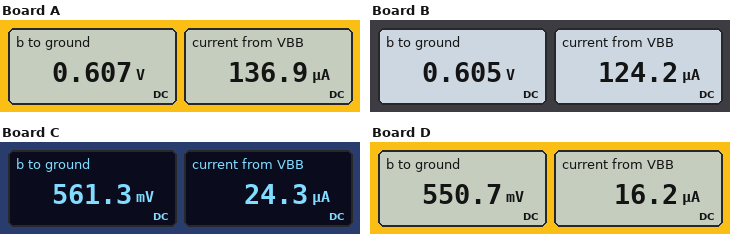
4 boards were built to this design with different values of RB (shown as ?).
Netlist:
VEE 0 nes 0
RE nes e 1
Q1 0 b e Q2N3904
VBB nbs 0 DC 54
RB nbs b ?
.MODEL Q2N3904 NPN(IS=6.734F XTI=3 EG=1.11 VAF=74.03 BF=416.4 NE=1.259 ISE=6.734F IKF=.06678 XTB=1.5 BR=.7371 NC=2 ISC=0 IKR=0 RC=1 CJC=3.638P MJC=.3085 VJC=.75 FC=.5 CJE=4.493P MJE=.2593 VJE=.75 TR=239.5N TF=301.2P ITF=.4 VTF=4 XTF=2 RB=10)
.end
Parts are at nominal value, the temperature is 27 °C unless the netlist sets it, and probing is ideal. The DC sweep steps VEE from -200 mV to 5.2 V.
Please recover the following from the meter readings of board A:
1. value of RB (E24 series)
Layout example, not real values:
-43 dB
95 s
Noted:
390 kΩ
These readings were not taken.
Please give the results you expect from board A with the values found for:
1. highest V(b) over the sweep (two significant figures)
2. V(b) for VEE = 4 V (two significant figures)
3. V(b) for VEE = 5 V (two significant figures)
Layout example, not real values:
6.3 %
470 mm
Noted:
610 mV
-3.2 V
-4.2 V
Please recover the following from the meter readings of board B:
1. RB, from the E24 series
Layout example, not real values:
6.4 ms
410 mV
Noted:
430 kΩ
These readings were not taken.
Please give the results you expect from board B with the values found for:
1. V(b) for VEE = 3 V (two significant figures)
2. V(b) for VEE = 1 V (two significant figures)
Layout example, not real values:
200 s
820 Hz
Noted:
-2.2 V
-230 mV
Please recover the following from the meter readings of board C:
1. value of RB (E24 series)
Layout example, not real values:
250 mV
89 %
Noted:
2.2 MΩ
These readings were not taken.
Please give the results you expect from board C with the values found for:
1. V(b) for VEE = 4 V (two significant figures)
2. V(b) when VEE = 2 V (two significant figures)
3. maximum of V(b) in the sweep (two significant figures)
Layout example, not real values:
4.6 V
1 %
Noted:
-3.3 V
-1.3 V
560 mV
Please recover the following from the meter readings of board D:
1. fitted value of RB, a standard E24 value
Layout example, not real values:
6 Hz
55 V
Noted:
3.3 MΩ
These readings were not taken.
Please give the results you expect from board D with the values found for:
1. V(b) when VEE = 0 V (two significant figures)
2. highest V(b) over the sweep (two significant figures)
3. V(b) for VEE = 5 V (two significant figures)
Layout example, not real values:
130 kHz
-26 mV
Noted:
550 mV
550 mV
-4.3 V
